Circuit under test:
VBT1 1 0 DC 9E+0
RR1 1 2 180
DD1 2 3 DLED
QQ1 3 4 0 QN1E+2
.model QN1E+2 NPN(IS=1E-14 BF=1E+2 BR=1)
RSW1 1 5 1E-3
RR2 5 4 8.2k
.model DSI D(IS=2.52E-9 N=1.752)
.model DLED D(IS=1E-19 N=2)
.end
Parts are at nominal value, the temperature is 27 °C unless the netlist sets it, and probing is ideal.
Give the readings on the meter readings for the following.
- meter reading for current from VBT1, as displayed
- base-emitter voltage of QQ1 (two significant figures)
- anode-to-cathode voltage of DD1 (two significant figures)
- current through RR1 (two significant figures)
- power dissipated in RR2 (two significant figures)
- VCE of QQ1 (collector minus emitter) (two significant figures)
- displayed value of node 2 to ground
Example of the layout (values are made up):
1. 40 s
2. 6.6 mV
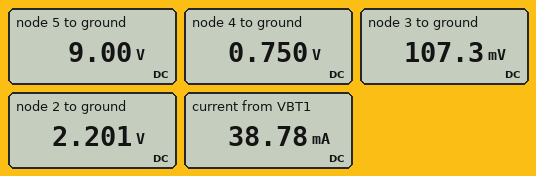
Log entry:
1. 38.78 mA
2. 750 mV
3. 2.1 V
4. 38 mA
5. 8.3 mW
6. 110 mV
7. 2.201 V
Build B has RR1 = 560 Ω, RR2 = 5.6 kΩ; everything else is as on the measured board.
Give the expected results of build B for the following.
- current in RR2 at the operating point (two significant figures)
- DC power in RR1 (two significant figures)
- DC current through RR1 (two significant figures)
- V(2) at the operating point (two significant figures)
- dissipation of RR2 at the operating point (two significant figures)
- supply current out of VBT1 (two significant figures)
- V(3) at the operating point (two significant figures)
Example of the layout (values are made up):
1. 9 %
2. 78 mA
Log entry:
1. 1.5 mA
2. 85 mW
3. 12 mA
4. 2.1 V
5. 12 mW
6. 14 mA
7. 63 mV
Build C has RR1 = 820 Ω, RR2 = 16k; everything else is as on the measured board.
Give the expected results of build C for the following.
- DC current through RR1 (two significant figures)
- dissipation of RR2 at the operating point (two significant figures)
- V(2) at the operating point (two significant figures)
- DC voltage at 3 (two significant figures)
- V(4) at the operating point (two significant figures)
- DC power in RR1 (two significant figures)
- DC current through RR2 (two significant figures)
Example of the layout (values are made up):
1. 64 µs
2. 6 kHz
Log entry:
1. 8.4 mA
2. 4.3 mW
3. 2.1 V
4. 80 mV
5. 710 mV
6. 58 mW
7. 520 µA
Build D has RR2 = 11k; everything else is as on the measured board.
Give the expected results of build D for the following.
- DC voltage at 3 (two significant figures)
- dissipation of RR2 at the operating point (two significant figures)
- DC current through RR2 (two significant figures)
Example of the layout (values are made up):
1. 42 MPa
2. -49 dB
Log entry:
1. 120 mV
2. 6.2 mW
3. 750 µA
